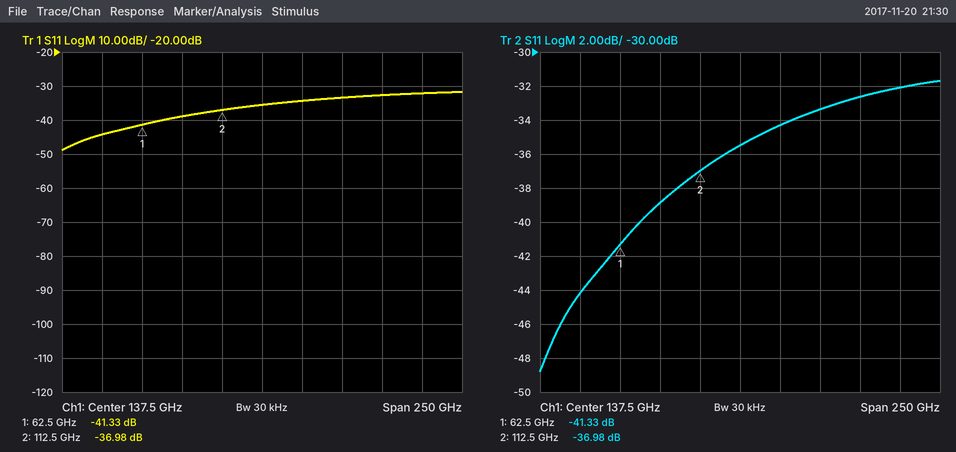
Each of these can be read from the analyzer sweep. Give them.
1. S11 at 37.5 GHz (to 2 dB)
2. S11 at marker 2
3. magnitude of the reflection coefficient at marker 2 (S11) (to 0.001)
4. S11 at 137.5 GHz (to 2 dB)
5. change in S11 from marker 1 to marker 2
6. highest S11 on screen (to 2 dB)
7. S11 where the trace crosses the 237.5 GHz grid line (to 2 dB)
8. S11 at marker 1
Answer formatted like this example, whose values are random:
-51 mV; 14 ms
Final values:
-44 dB; -36.98 dB; 0.014; -36 dB; 4.35 dB; -32 dB; -32 dB; -41.33 dB
